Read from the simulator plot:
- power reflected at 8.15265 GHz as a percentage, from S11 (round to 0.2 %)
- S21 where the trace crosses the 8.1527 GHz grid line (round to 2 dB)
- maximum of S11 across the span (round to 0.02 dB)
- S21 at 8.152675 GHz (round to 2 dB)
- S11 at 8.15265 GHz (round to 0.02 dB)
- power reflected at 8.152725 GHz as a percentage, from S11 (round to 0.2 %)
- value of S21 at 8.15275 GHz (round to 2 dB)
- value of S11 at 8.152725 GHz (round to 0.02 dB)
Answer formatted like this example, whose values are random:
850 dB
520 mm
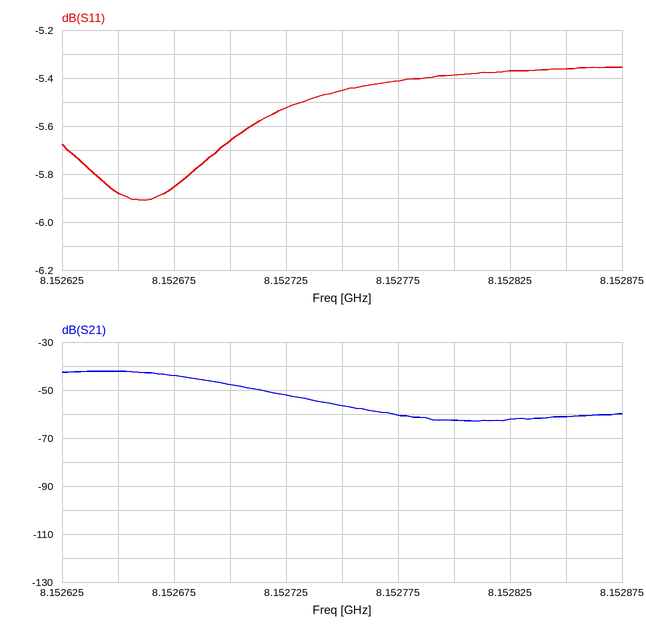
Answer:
25.8 %
-48 dB
-5.36 dB
-44 dB
-5.88 dB
28.0 %
-56 dB
-5.52 dB
